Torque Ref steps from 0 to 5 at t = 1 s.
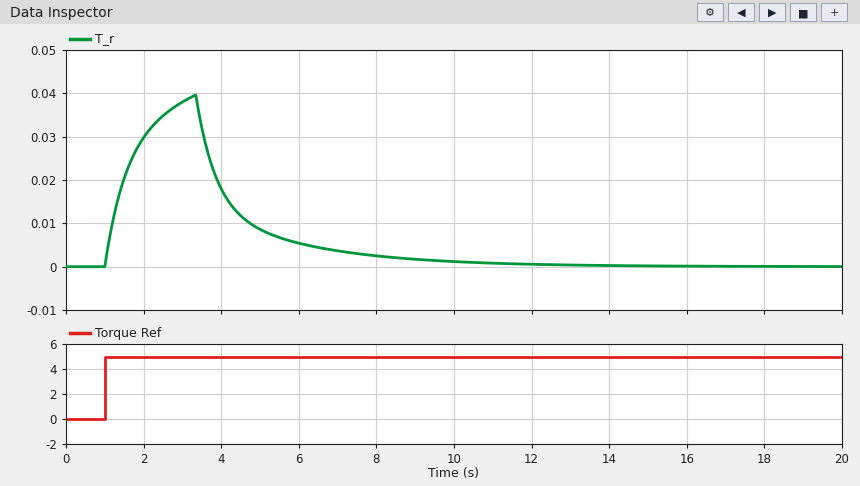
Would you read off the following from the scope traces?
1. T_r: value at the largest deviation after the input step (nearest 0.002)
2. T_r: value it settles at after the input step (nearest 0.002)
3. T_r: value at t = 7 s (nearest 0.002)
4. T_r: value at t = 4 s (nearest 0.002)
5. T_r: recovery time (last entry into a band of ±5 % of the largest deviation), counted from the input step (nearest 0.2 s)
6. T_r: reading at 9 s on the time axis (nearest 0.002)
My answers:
0.040
0.000
0.004
0.018
7.6 s
0.002
